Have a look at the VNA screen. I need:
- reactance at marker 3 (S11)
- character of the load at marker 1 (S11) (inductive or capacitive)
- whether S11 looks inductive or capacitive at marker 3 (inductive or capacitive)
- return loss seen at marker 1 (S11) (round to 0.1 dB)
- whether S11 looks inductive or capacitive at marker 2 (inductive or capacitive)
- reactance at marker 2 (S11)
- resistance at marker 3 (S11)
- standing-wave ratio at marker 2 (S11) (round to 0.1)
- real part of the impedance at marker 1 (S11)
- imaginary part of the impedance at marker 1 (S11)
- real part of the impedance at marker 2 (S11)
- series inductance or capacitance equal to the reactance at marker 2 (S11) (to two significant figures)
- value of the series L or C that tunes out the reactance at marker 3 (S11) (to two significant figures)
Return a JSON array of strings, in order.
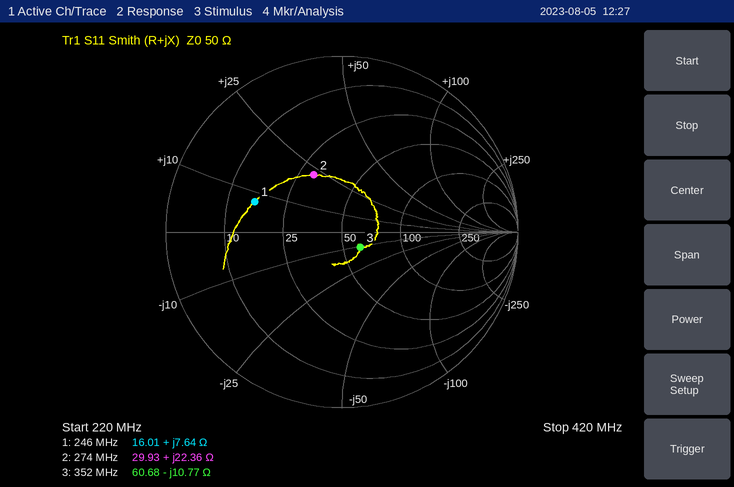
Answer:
["-10.77 Ω", "inductive", "capacitive", "5.6 dB", "inductive", "+22.36 Ω", "60.68 Ω", "2.1", "16.01 Ω", "+7.64 Ω", "29.93 Ω", "13 nH", "4.9 nH"]
